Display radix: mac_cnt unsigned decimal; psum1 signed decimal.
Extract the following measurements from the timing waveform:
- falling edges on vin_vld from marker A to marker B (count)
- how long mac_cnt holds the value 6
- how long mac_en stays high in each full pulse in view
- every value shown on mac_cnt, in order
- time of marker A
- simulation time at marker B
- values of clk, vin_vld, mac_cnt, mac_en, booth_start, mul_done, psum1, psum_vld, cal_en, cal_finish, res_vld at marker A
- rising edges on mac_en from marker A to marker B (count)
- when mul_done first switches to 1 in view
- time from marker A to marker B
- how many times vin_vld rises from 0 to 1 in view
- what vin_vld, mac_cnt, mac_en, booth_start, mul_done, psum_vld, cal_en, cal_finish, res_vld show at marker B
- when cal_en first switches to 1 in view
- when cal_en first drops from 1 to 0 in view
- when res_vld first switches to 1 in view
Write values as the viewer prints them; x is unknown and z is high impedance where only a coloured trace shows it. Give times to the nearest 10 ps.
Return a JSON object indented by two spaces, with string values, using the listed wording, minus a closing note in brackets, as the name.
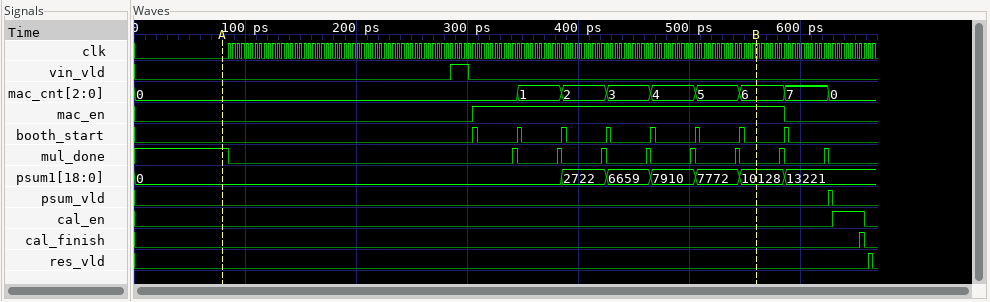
{
  "falling edges on vin_vld from marker A to marker B": "1",
  "how long mac_cnt holds the value 6": "40 ps",
  "how long mac_en stays high in each full pulse in view": "280 ps",
  "every value shown on mac_cnt, in order": "0, 1, 2, 3, 4, 5, 6, 7, 0",
  "time of marker A": "80 ps",
  "simulation time at marker B": "560 ps",
  "values of clk, vin_vld, mac_cnt, mac_en, booth_start, mul_done, psum1, psum_vld, cal_en, cal_finish, res_vld at marker A": "clk=0, vin_vld=0, mac_cnt=0, mac_en=0, booth_start=0, mul_done=1, psum1=0, psum_vld=0, cal_en=0, cal_finish=0, res_vld=0",
  "rising edges on mac_en from marker A to marker B": "1",
  "when mul_done first switches to 1 in view": "340 ps",
  "time from marker A to marker B": "480 ps",
  "how many times vin_vld rises from 0 to 1 in view": "1",
  "what vin_vld, mac_cnt, mac_en, booth_start, mul_done, psum_vld, cal_en, cal_finish, res_vld show at marker B": "vin_vld=0, mac_cnt=6, mac_en=1, booth_start=0, mul_done=0, psum_vld=0, cal_en=0, cal_finish=0, res_vld=0",
  "when cal_en first switches to 1 in view": "630 ps",
  "when cal_en first drops from 1 to 0 in view": "660 ps",
  "when res_vld first switches to 1 in view": "660 ps"
}
